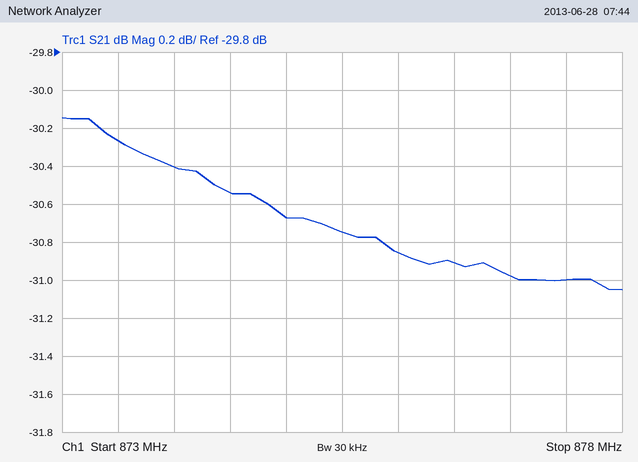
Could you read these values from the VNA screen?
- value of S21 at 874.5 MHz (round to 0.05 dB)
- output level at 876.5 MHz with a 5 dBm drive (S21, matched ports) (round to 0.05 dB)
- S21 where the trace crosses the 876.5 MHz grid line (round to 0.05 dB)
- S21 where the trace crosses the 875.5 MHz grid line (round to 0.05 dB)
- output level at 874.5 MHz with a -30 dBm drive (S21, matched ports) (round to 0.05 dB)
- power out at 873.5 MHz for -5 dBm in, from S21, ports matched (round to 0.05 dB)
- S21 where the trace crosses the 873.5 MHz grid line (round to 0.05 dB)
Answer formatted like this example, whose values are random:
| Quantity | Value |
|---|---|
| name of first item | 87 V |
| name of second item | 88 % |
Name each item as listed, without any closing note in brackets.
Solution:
| Quantity | Value |
|---|---|
| value of S21 at 874.5 MHz | -30.55 dB |
| output level at 876.5 MHz with a 5 dBm drive (S21, matched ports) | -25.90 dBm |
| S21 where the trace crosses the 876.5 MHz grid line | -30.90 dB |
| S21 where the trace crosses the 875.5 MHz grid line | -30.75 dB |
| output level at 874.5 MHz with a -30 dBm drive (S21, matched ports) | -60.55 dBm |
| power out at 873.5 MHz for -5 dBm in, from S21, ports matched | -35.25 dBm |
| S21 where the trace crosses the 873.5 MHz grid line | -30.25 dB |
